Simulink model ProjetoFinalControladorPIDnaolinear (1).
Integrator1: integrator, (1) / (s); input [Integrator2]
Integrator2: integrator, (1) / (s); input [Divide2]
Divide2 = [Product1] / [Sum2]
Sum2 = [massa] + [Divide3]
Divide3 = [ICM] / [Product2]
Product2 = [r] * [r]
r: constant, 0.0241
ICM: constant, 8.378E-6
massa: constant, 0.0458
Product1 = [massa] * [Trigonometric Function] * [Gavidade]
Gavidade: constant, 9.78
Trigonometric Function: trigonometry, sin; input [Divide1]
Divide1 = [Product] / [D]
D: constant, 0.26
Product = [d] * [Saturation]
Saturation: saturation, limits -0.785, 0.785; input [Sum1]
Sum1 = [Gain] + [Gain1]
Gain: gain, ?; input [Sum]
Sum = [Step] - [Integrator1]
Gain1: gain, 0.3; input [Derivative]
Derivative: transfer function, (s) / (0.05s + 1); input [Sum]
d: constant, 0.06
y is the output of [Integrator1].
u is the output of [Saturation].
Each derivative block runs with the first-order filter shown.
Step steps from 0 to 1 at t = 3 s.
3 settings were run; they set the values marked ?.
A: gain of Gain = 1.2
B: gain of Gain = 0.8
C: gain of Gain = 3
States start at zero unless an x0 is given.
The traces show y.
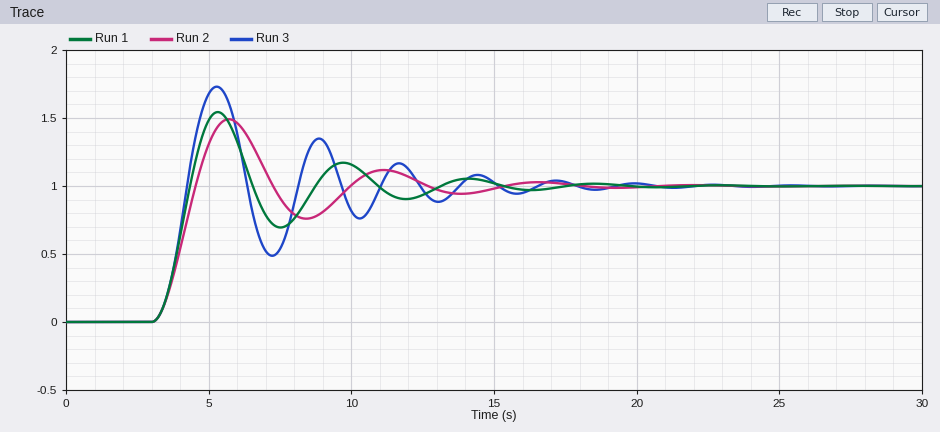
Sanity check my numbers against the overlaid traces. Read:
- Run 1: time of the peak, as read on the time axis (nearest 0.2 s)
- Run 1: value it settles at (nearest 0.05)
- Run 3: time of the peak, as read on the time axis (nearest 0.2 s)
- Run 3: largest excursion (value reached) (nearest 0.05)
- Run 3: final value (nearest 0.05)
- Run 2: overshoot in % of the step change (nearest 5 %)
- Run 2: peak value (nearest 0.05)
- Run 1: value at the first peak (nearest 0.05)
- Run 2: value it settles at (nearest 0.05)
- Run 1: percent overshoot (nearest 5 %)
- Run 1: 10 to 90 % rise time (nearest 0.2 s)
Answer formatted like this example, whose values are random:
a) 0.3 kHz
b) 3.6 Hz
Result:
a) 5.4 s
b) 1.00
c) 5.2 s
d) 1.75
e) 1.00
f) 50 %
g) 1.50
h) 1.55
i) 1.00
j) 55 %
k) 0.8 s
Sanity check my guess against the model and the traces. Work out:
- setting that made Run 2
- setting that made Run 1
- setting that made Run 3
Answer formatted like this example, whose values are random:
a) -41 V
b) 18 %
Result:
a) B
b) A
c) C
